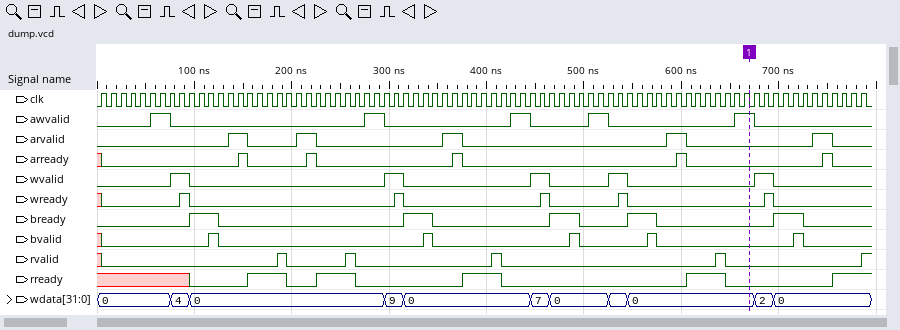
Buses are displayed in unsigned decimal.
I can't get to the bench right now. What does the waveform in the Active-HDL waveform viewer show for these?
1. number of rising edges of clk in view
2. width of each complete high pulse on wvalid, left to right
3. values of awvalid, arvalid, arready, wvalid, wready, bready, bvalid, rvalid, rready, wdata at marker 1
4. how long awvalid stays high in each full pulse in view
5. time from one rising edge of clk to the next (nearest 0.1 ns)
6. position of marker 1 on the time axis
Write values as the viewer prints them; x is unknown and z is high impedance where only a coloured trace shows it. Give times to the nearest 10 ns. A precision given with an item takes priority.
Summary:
79
20 ns, 20 ns, 20 ns, 20 ns, 20 ns
awvalid=1, arvalid=0, arready=0, wvalid=0, wready=0, bready=0, bvalid=0, rvalid=0, rready=0, wdata=0
20 ns, 20 ns, 20 ns, 20 ns, 20 ns
10 ns
670 ns
